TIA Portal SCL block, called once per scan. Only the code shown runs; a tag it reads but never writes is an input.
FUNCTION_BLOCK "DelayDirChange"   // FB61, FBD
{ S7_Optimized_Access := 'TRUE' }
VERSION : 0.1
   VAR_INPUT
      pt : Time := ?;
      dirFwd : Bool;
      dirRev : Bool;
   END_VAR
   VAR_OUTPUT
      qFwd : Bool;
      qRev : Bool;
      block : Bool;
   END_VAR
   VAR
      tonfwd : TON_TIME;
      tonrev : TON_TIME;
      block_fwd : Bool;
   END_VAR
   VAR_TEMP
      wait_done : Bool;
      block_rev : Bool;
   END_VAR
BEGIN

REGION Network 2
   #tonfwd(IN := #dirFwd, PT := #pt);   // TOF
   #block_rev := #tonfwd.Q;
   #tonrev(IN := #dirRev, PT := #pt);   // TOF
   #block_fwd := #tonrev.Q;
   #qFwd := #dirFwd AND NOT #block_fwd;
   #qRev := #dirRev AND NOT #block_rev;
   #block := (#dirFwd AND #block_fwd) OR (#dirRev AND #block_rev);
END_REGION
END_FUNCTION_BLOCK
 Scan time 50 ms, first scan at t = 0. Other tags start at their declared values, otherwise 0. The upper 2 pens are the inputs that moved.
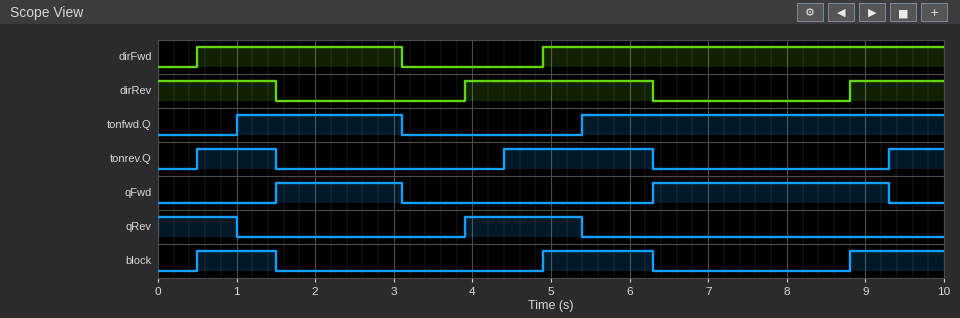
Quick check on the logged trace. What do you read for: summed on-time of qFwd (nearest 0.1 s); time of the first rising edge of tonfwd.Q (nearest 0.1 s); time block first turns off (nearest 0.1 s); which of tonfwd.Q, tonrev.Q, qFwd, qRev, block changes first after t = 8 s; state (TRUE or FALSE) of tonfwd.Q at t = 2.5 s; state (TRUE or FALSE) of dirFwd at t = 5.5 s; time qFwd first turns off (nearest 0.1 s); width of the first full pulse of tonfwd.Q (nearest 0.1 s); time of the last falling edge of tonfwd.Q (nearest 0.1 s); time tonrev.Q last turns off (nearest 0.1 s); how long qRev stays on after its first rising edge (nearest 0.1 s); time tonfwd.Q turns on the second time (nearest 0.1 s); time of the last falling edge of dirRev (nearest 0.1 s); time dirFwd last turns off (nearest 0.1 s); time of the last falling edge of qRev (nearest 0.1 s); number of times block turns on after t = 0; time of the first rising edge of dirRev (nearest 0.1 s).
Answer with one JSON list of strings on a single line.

["4.6 s", "1.0 s", "1.5 s", "block", "TRUE", "TRUE", "3.1 s", "2.1 s", "3.1 s", "6.3 s", "1.5 s", "5.4 s", "6.3 s", "3.1 s", "5.4 s", "3", "3.9 s"]
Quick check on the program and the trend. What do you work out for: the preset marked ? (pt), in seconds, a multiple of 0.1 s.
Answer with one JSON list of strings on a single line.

["0.5 s"]
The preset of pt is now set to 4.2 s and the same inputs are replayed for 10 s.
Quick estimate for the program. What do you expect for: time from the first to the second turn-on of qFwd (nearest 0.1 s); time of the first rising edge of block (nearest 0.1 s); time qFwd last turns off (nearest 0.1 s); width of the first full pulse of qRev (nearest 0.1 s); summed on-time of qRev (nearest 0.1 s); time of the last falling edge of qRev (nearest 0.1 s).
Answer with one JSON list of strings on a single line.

["4.4 s", "9.1 s", "3.1 s", "2.4 s", "4.2 s", "9.1 s"]
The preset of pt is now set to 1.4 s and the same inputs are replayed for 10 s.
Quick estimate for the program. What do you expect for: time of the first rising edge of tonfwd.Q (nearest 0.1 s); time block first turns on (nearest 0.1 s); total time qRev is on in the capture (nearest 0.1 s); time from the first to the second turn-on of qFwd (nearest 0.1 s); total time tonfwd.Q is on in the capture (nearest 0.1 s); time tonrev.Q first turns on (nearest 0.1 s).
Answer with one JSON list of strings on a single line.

["1.9 s", "1.4 s", "3.9 s", "1.0 s", "4.9 s", "1.4 s"]
